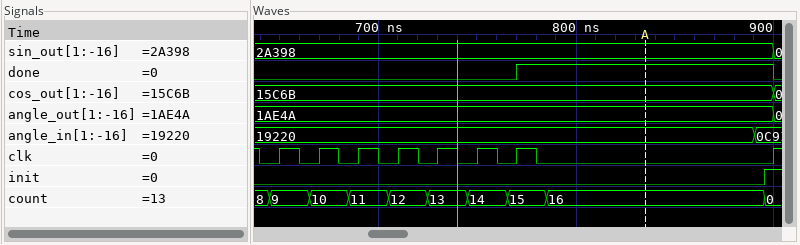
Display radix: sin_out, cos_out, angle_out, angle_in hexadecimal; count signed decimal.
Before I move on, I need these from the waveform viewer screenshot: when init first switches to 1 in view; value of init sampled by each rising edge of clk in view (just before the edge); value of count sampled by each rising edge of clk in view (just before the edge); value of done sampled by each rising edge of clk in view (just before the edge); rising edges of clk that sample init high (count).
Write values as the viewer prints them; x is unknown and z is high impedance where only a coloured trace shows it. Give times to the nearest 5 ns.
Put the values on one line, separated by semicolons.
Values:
895 ns; 0 0 0 0 0 0 0 1; 9, 10, 11, 12, 13, 14, 15, 0; 0 0 0 0 0 0 0 1; 1
